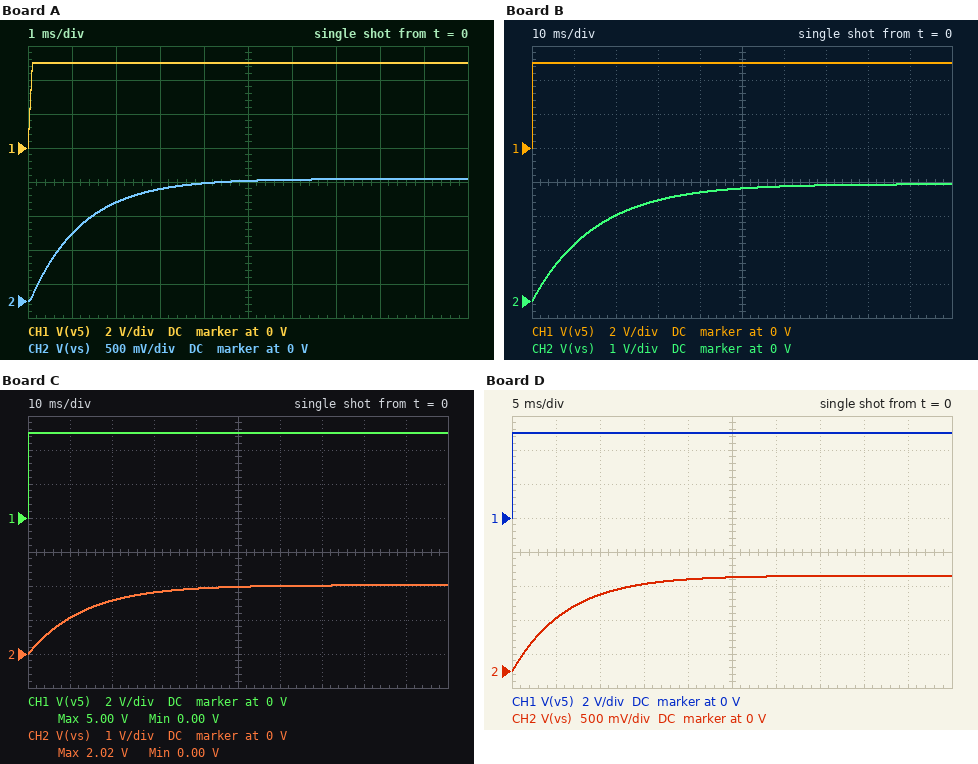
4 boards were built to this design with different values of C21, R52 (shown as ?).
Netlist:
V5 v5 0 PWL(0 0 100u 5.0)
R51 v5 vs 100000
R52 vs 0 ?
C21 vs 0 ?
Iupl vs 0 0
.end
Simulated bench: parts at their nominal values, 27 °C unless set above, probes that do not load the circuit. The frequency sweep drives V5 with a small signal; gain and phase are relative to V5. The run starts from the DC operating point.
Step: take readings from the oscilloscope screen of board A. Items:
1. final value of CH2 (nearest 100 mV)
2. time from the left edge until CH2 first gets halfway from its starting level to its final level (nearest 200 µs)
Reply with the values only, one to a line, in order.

1.8 V
800 µs
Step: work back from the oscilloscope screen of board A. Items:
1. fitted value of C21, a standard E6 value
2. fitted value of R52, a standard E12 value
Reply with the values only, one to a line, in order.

33 nF
56 kΩ
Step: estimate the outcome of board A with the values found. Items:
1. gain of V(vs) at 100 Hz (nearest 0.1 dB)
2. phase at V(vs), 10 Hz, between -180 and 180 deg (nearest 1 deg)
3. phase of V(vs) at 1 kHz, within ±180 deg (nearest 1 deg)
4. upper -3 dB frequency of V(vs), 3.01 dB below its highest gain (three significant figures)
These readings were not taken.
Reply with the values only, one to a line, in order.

-10.8 dB
-4 deg
-82 deg
134 Hz
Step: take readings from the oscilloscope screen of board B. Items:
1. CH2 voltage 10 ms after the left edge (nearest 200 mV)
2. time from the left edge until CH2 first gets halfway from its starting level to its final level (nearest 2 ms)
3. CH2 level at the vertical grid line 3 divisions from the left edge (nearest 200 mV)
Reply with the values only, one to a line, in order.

1.6 V
10 ms
3.0 V
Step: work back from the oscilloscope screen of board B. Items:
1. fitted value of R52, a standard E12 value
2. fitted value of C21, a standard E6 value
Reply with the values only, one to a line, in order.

220 kΩ
220 nF
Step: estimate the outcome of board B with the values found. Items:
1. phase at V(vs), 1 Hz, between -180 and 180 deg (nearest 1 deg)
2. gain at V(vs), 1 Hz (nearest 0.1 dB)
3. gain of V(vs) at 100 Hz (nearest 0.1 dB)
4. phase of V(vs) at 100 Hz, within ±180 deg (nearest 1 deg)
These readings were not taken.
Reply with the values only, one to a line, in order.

-5 deg
-3.3 dB
-22.9 dB
-84 deg
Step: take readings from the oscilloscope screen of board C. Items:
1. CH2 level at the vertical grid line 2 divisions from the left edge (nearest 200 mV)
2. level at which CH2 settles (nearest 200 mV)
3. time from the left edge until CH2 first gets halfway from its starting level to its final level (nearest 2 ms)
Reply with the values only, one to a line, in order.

1.6 V
2.0 V
10 ms
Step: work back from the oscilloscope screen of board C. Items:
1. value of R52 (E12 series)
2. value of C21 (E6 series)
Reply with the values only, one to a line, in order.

68 kΩ
330 nF
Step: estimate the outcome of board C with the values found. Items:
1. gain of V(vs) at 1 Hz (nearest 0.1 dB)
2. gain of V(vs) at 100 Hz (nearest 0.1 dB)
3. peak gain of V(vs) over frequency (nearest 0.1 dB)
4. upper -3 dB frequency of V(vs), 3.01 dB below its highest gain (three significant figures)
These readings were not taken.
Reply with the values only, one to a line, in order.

-7.9 dB
-26.4 dB
-7.9 dB
11.9 Hz
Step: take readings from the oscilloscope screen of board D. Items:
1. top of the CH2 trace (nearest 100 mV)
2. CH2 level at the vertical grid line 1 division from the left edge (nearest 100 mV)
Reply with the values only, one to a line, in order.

1.4 V
800 mV
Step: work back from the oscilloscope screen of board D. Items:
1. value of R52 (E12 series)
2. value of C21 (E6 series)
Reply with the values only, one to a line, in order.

39 kΩ
220 nF
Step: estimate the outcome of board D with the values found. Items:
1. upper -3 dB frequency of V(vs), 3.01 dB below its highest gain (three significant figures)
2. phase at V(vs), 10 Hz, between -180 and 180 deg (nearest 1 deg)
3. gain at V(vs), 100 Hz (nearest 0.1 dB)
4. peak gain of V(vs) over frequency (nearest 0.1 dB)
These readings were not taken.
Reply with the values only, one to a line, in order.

25.8 Hz
-21 deg
-23.1 dB
-11.0 dB
